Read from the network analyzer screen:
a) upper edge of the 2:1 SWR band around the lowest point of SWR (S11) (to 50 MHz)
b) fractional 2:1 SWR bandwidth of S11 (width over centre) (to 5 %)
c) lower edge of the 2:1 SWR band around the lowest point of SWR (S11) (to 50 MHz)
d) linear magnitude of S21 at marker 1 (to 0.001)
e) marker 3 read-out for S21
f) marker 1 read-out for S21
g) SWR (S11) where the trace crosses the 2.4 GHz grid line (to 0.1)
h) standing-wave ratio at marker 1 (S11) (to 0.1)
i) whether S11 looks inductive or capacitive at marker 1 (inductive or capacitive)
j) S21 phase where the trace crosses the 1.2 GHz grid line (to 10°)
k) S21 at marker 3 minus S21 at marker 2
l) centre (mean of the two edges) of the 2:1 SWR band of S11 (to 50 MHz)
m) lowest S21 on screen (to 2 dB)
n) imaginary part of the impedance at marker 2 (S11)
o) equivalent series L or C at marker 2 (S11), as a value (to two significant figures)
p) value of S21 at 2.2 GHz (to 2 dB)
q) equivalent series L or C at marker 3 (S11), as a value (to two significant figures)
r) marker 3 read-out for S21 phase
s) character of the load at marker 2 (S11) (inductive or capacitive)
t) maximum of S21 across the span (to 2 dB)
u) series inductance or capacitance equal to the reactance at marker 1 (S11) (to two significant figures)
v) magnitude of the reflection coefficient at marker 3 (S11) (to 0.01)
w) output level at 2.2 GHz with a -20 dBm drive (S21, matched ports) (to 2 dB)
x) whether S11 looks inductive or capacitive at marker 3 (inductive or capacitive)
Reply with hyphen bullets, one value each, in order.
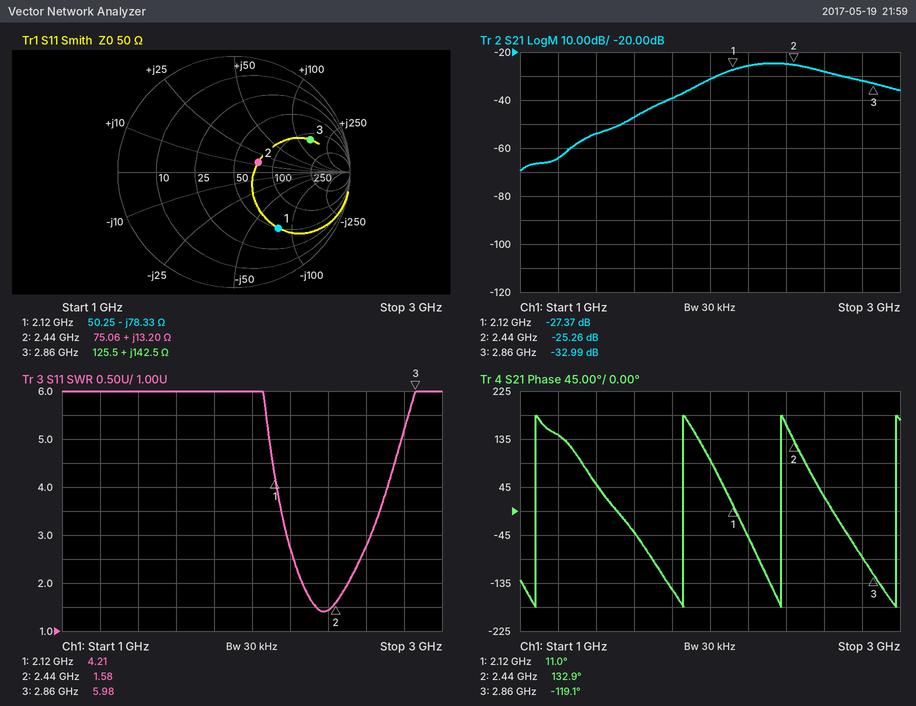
- 2.50 GHz
- 10 %
- 2.25 GHz
- 0.043
- -32.99 dB
- -27.37 dB
- 1.4
- 4.2
- capacitive
- 140°
- -7.73 dB
- 2.40 GHz
- -70 dB
- +13.20 Ω
- 860 pH
- -26 dB
- 7.9 nH
- -119.1°
- inductive
- -24 dB
- 960 fF
- 0.71
- -46 dBm
- inductive
